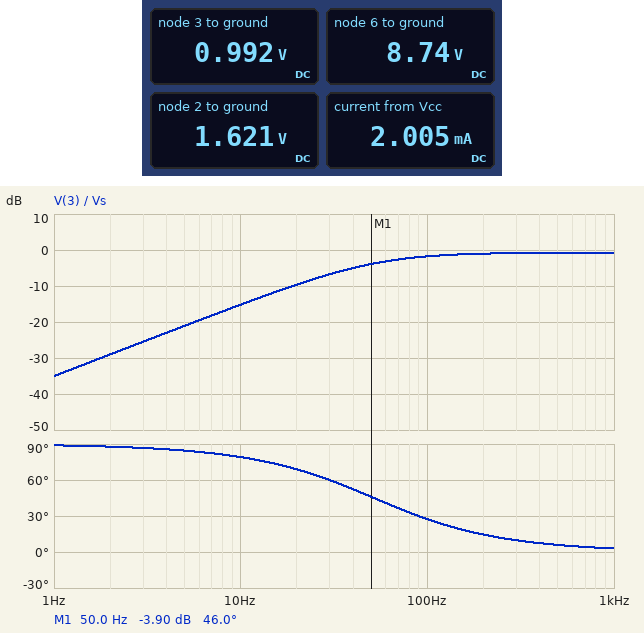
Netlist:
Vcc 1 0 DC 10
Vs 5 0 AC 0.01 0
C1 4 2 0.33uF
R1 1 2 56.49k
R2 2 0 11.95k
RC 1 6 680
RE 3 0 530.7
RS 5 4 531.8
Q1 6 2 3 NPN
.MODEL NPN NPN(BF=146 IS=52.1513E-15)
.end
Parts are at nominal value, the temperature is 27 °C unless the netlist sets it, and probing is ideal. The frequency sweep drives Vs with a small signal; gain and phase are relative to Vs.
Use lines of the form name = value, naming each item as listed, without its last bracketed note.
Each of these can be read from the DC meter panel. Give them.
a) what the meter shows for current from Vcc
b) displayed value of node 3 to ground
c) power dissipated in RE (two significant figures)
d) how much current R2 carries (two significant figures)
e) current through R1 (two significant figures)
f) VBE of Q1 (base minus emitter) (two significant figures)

what the meter shows for current from Vcc = 2.005 mA
displayed value of node 3 to ground = 0.992 V
power dissipated in RE = 1.9 mW
how much current R2 carries = 140 µA
current through R1 = 150 µA
VBE of Q1 (base minus emitter) = 630 mV
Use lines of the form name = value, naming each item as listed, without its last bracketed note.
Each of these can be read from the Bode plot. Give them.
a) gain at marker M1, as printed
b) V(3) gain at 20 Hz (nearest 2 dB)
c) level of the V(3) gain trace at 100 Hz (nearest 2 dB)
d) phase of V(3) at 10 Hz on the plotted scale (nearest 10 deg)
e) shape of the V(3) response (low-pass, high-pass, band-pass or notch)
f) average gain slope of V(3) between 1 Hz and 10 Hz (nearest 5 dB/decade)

gain at marker M1, as printed = -3.90 dB
V(3) gain at 20 Hz = -10 dB
level of the V(3) gain trace at 100 Hz = -2 dB
phase of V(3) at 10 Hz on the plotted scale = 80 deg
shape of the V(3) response = high-pass
average gain slope of V(3) between 1 Hz and 10 Hz = 20 dB/decade
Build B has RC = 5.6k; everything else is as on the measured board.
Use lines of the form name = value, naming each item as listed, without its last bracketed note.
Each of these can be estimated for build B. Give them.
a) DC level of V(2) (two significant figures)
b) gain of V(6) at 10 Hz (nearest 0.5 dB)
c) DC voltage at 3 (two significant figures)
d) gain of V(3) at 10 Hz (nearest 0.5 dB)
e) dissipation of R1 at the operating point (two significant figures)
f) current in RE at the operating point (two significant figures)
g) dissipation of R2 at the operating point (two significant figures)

DC level of V(2) = 1.5 V
gain of V(6) at 10 Hz = -33.5 dB
DC voltage at 3 = 870 mV
gain of V(3) at 10 Hz = -38.0 dB
dissipation of R1 at the operating point = 1.3 mW
current in RE at the operating point = 1.6 mA
dissipation of R2 at the operating point = 190 µW
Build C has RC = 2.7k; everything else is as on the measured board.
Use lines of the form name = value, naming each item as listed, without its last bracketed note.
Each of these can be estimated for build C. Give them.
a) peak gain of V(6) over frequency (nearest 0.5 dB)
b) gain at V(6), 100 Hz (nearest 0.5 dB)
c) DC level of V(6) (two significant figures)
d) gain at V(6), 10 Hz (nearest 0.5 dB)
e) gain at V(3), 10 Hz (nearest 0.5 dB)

peak gain of V(6) over frequency = 13.5 dB
gain at V(6), 100 Hz = 12.5 dB
DC level of V(6) = 5.0 V
gain at V(6), 10 Hz = -1.0 dB
gain at V(3), 10 Hz = -15.0 dB
